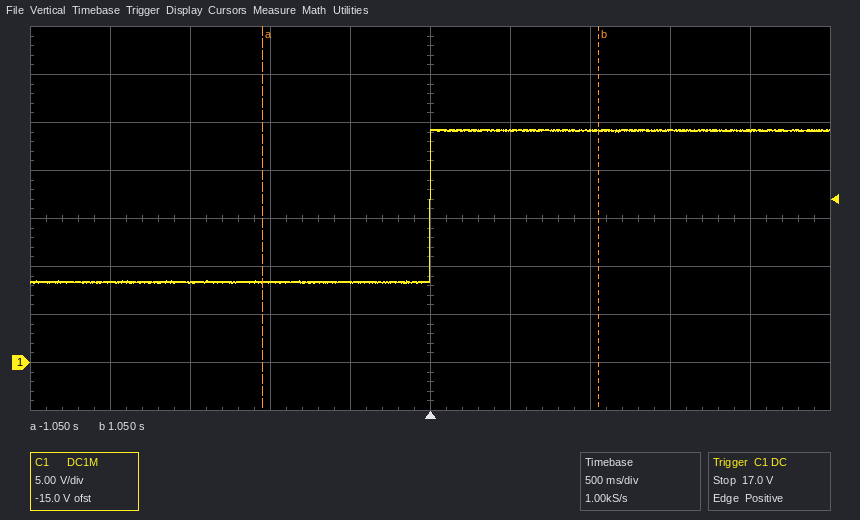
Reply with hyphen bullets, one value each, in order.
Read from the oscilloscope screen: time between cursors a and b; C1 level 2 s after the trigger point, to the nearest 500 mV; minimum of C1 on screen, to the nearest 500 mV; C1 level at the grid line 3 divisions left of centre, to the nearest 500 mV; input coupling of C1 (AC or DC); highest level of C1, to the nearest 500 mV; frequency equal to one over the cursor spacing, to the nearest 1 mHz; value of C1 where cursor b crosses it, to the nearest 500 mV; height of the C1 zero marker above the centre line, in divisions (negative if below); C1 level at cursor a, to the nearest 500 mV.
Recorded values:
- 2.10 s
- 24.0 V
- 8.0 V
- 8.5 V
- DC
- 24.5 V
- 476 mHz
- 24.0 V
- -3.0 div
- 8.5 V
